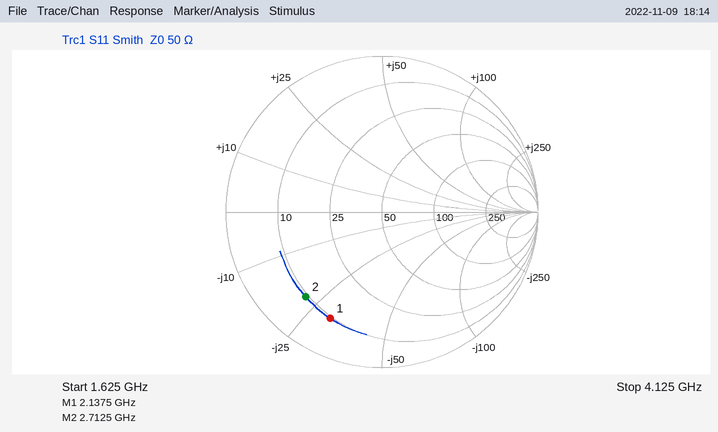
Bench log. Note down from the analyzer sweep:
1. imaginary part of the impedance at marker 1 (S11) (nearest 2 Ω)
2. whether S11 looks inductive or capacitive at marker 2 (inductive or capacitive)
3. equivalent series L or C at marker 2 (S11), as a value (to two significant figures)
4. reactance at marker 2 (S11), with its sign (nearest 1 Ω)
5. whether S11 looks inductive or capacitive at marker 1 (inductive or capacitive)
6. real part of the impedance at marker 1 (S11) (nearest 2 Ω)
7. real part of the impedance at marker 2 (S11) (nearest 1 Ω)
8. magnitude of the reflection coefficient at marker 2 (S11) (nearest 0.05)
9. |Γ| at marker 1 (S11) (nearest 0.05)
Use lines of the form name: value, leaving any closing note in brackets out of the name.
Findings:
imaginary part of the impedance at marker 1 (S11): -30 Ω
whether S11 looks inductive or capacitive at marker 2: capacitive
equivalent series L or C at marker 2 (S11), as a value: 2.7 pF
reactance at marker 2 (S11), with its sign: -22 Ω
whether S11 looks inductive or capacitive at marker 1: capacitive
real part of the impedance at marker 1 (S11): 10 Ω
real part of the impedance at marker 2 (S11): 9 Ω
magnitude of the reflection coefficient at marker 2 (S11): 0.75
|Γ| at marker 1 (S11): 0.75
